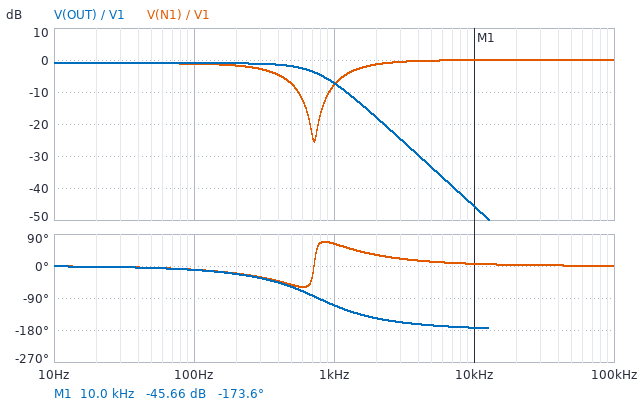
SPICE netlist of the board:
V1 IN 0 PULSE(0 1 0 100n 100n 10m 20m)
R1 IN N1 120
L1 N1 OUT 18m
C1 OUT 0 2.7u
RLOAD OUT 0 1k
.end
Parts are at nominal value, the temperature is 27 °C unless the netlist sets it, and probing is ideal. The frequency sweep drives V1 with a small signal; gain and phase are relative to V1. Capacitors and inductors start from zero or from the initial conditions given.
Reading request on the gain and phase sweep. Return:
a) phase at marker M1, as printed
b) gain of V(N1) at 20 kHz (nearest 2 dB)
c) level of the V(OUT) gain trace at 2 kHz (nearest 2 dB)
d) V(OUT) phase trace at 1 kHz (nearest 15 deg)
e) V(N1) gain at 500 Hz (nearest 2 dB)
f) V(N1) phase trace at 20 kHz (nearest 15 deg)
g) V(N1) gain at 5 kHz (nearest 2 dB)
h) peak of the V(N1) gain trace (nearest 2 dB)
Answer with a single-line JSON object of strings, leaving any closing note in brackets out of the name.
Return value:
{"phase at marker M1, as printed": "-173.6 deg", "gain of V(N1) at 20 kHz": "0 dB", "level of the V(OUT) gain trace at 2 kHz": "-18 dB", "V(OUT) phase trace at 1 kHz": "-105 deg", "V(N1) gain at 500 Hz": "-8 dB", "V(N1) phase trace at 20 kHz": "0 deg", "V(N1) gain at 5 kHz": "0 dB", "peak of the V(N1) gain trace": "0 dB"}
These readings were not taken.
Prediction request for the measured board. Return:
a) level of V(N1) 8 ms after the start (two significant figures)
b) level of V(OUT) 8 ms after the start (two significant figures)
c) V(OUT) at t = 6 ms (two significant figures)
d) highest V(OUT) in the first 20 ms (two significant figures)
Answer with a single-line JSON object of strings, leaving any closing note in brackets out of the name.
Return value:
{"level of V(N1) 8 ms after the start": "890 mV", "level of V(OUT) 8 ms after the start": "890 mV", "V(OUT) at t = 6 ms": "890 mV", "highest V(OUT) in the first 20 ms": "920 mV"}
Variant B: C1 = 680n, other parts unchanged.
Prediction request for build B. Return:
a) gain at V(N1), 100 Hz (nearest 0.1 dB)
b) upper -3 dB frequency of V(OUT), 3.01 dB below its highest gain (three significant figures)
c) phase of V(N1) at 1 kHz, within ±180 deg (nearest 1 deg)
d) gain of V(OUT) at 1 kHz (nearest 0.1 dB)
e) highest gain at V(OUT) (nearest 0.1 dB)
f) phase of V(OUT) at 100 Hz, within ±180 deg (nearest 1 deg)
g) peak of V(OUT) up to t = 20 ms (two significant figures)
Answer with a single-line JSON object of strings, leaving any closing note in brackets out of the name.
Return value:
{"gain at V(N1), 100 Hz": "-1.0 dB", "upper -3 dB frequency of V(OUT), 3.01 dB below its highest gain": "1.81 kHz", "phase of V(N1) at 1 kHz, within ±180 deg": "-32 deg", "gain of V(OUT) at 1 kHz": "1.0 dB", "highest gain at V(OUT)": "1.3 dB", "phase of V(OUT) at 100 Hz, within ±180 deg": "-3 deg", "peak of V(OUT) up to t = 20 ms": "1.1 V"}
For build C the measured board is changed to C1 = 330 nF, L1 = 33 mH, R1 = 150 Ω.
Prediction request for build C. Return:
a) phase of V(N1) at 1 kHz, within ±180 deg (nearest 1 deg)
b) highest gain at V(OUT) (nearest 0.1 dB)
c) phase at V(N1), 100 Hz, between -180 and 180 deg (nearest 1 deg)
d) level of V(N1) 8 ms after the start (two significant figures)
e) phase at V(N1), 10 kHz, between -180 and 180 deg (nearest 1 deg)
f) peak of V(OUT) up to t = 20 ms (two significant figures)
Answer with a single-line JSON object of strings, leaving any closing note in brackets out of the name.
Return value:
{"phase of V(N1) at 1 kHz, within ±180 deg": "-16 deg", "highest gain at V(OUT)": "2.1 dB", "phase at V(N1), 100 Hz, between -180 and 180 deg": "-1 deg", "level of V(N1) 8 ms after the start": "870 mV", "phase at V(N1), 10 kHz, between -180 and 180 deg": "4 deg", "peak of V(OUT) up to t = 20 ms": "1.1 V"}
